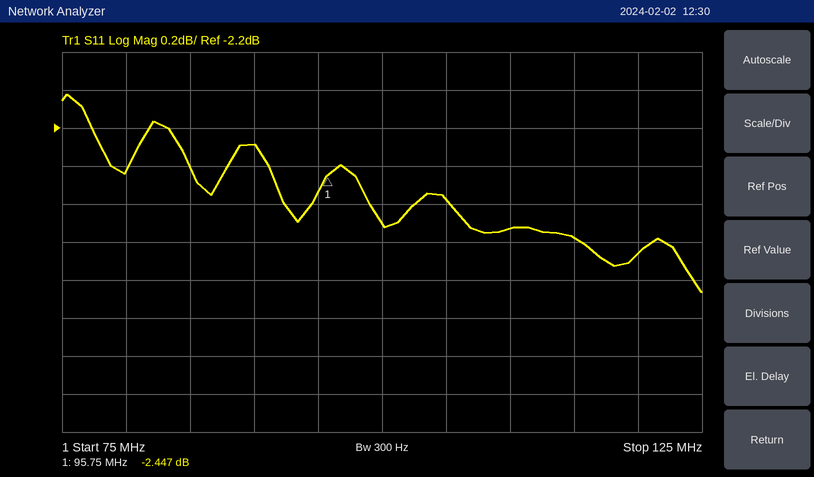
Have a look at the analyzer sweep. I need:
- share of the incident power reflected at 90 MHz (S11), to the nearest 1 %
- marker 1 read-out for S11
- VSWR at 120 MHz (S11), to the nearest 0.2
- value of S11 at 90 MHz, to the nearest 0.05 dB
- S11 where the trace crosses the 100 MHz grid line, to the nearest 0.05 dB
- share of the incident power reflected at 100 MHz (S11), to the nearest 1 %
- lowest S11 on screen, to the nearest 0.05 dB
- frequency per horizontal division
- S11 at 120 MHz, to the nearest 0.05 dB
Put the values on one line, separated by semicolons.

59 %; -2.447 dB; 6.2; -2.30 dB; -2.70 dB; 54 %; -3.05 dB; 5 MHz; -2.85 dB
